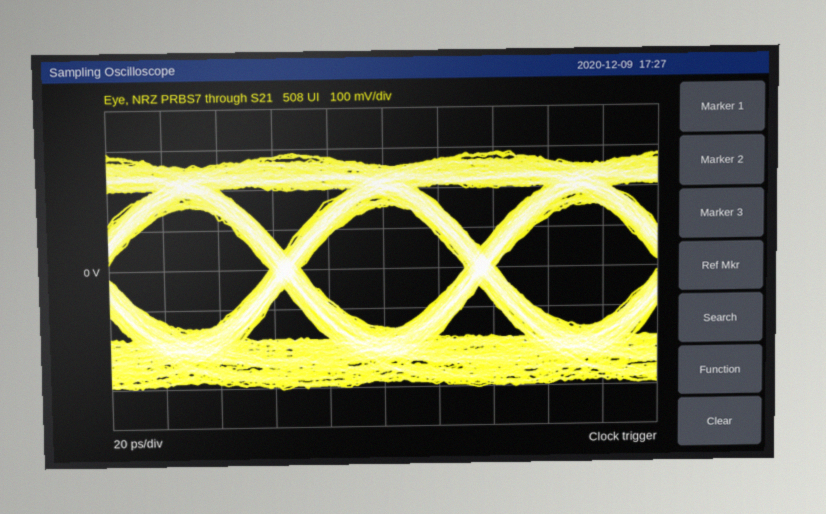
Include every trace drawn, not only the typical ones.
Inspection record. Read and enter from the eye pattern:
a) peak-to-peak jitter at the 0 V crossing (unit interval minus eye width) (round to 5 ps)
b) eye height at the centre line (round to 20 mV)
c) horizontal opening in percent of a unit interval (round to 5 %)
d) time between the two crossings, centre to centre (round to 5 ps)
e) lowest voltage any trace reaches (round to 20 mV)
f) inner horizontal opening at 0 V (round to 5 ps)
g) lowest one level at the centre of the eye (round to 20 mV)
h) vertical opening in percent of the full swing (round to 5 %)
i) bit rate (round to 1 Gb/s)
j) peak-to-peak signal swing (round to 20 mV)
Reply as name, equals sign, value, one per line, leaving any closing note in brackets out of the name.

peak-to-peak jitter at the 0 V crossing (unit interval minus eye width) = 10 ps
eye height at the centre line = 300 mV
horizontal opening in percent of a unit interval = 85 %
time between the two crossings, centre to centre = 70 ps
lowest voltage any trace reaches = -300 mV
inner horizontal opening at 0 V = 60 ps
lowest one level at the centre of the eye = 160 mV
vertical opening in percent of the full swing = 50 %
bit rate = 14 Gb/s
peak-to-peak signal swing = 600 mV
